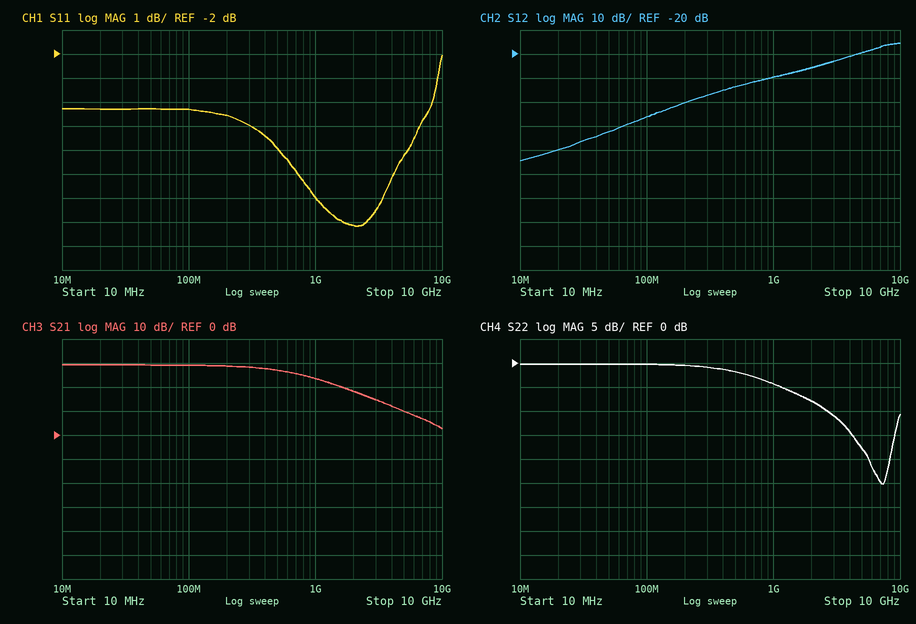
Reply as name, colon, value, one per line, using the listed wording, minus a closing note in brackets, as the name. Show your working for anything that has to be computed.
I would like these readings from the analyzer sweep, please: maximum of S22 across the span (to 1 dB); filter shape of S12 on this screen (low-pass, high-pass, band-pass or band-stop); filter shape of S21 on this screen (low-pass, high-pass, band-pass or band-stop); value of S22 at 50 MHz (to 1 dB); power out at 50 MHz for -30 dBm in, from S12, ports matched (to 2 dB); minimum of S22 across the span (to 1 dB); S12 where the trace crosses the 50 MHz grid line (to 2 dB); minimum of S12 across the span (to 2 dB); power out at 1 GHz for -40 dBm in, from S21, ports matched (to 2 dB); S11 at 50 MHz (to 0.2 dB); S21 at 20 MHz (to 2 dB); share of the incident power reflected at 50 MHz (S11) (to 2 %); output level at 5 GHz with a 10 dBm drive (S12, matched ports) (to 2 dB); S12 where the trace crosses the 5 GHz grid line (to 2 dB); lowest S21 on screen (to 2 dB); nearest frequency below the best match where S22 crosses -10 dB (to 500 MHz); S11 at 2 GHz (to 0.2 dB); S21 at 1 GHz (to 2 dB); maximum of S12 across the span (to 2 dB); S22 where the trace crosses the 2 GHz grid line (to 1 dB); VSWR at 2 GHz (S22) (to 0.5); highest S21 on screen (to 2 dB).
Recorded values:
maximum of S22 across the span: 0 dB
filter shape of S12 on this screen: high-pass
filter shape of S21 on this screen: low-pass
value of S22 at 50 MHz: 0 dB
power out at 50 MHz for -30 dBm in, from S12, ports matched: -30 dBm + (-52 dB) = -82 dBm
minimum of S22 across the span: -25 dB
S12 where the trace crosses the 50 MHz grid line: -52 dB
minimum of S12 across the span: -64 dB
power out at 1 GHz for -40 dBm in, from S21, ports matched: -40 dBm + (24 dB) = -16 dBm
S11 at 50 MHz: -4.2 dB
S21 at 20 MHz: 30 dB
share of the incident power reflected at 50 MHz (S11): 10^(-4.2/10) ≈ 38 %
output level at 5 GHz with a 10 dBm drive (S12, matched ports): 10 dBm + (-20 dB) = -10 dBm
S12 where the trace crosses the 5 GHz grid line: -20 dB
lowest S21 on screen: 2 dB
nearest frequency below the best match where S22 crosses -10 dB: 2.5 GHz
S11 at 2 GHz: -9.2 dB
S21 at 1 GHz: 24 dB
maximum of S12 across the span: -16 dB
S22 where the trace crosses the 2 GHz grid line: -8 dB
VSWR at 2 GHz (S22): |Γ| = 10^(-8/20) = 0.3981; VSWR = (1 + 0.3981)/(1 − 0.3981) ≈ 2.32, so 2.5 to the nearest 0.5
highest S21 on screen: 30 dB
